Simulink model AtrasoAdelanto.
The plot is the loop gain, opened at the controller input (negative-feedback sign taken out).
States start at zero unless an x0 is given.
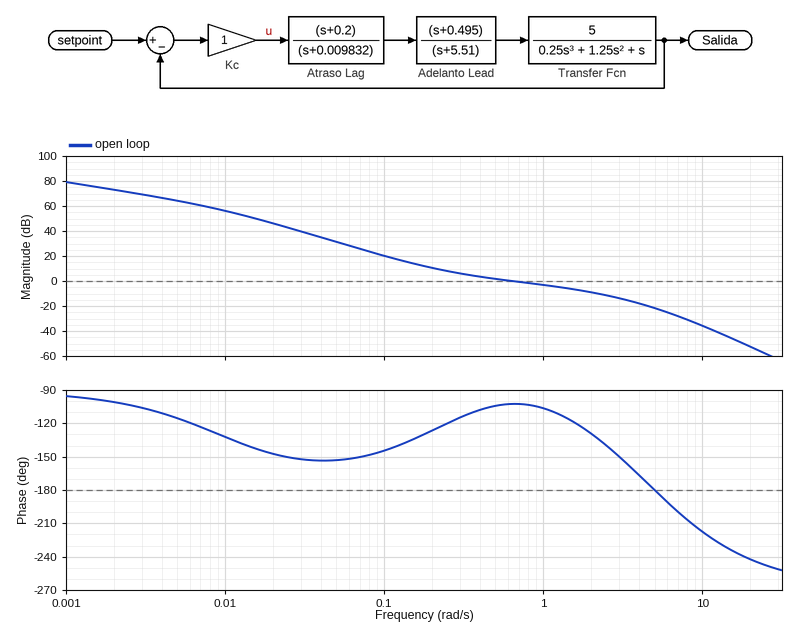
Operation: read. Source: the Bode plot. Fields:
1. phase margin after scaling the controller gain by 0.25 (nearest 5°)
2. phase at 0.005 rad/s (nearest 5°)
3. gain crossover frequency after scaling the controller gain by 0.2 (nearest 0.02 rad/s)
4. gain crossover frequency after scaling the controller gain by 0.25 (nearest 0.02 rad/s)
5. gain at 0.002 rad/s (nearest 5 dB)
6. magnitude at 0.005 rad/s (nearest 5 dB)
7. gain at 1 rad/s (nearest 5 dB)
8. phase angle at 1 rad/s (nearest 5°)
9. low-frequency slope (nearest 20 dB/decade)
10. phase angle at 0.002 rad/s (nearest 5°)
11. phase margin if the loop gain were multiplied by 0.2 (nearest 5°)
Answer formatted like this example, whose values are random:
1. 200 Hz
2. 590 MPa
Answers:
1. 50°
2. -115°
3. 0.16 rad/s
4. 0.18 rad/s
5. 75 dB
6. 65 dB
7. -5 dB
8. -105°
9. -20 dB/decade
10. -100°
11. 45°
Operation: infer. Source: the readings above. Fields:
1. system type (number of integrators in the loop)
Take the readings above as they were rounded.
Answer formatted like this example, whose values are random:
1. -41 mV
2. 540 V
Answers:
1. 1
